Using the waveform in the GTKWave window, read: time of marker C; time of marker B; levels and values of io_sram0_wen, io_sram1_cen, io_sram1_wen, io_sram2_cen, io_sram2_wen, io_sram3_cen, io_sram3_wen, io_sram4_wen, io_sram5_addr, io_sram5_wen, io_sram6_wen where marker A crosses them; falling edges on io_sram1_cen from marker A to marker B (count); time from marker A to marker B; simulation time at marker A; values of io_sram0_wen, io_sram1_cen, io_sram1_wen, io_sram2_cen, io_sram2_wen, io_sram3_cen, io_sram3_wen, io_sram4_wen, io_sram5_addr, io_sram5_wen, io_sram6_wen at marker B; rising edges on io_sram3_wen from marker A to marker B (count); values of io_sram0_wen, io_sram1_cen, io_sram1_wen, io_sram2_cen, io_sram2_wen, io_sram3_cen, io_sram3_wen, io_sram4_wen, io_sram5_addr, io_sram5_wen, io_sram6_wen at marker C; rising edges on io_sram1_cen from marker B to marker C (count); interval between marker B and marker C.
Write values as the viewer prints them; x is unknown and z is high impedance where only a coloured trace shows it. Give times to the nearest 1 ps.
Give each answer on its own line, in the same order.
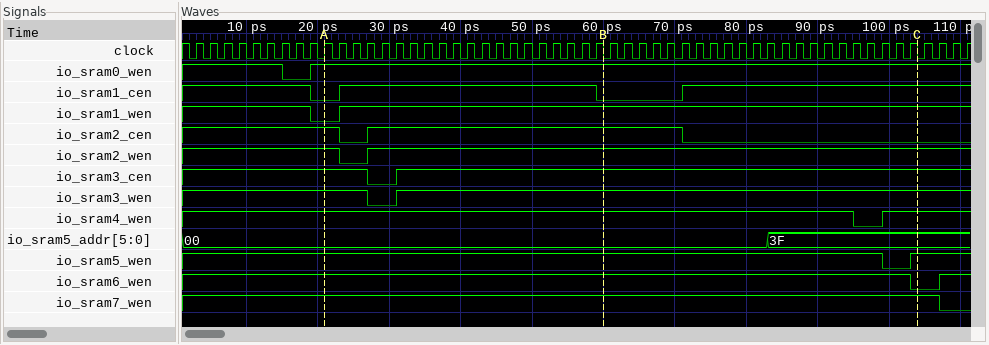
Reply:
104 ps
60 ps
io_sram0_wen=1, io_sram1_cen=0, io_sram1_wen=0, io_sram2_cen=1, io_sram2_wen=1, io_sram3_cen=1, io_sram3_wen=1, io_sram4_wen=1, io_sram5_addr=00, io_sram5_wen=1, io_sram6_wen=1
1
39 ps
21 ps
io_sram0_wen=1, io_sram1_cen=0, io_sram1_wen=1, io_sram2_cen=1, io_sram2_wen=1, io_sram3_cen=1, io_sram3_wen=1, io_sram4_wen=1, io_sram5_addr=00, io_sram5_wen=1, io_sram6_wen=1
1
io_sram0_wen=1, io_sram1_cen=1, io_sram1_wen=1, io_sram2_cen=0, io_sram2_wen=1, io_sram3_cen=1, io_sram3_wen=1, io_sram4_wen=1, io_sram5_addr=3F, io_sram5_wen=1, io_sram6_wen=0
1
44 ps
